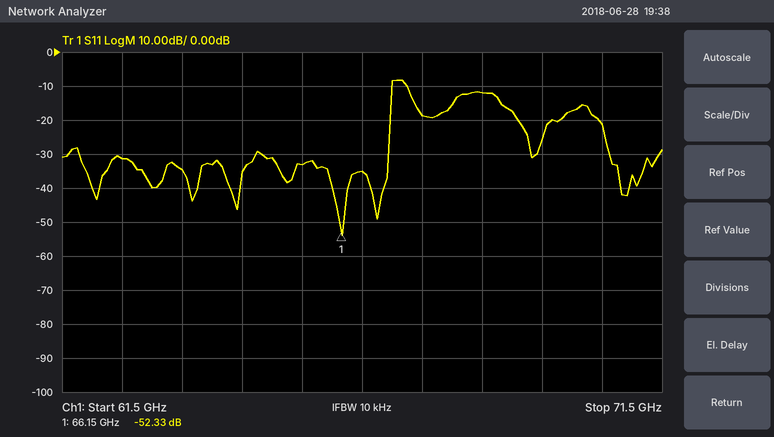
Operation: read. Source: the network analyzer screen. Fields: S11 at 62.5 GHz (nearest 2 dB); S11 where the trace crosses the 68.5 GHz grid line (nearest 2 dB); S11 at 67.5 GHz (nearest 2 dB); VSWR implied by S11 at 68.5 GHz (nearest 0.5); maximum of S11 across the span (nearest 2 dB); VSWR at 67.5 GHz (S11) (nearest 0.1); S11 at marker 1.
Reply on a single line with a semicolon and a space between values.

-32 dB; -12 dB; -18 dB; 1.5; -8 dB; 1.3; -52.33 dB
